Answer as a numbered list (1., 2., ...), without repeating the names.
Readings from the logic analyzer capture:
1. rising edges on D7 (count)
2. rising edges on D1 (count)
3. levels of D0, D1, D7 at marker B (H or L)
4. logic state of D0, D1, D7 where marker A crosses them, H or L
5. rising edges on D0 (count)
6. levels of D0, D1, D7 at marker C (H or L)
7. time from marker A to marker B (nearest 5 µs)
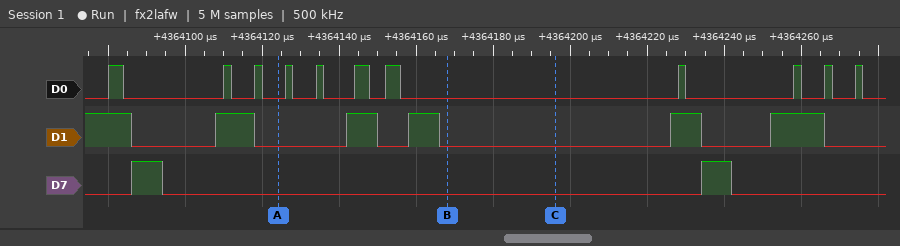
1. 2
2. 5
3. D0=L, D1=L, D7=L
4. D0=L, D1=L, D7=L
5. 11
6. D0=L, D1=L, D7=L
7. 45 µs
